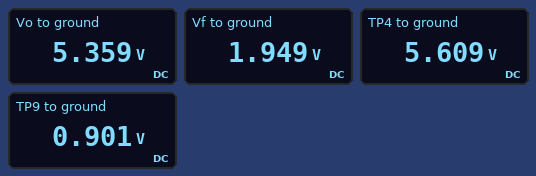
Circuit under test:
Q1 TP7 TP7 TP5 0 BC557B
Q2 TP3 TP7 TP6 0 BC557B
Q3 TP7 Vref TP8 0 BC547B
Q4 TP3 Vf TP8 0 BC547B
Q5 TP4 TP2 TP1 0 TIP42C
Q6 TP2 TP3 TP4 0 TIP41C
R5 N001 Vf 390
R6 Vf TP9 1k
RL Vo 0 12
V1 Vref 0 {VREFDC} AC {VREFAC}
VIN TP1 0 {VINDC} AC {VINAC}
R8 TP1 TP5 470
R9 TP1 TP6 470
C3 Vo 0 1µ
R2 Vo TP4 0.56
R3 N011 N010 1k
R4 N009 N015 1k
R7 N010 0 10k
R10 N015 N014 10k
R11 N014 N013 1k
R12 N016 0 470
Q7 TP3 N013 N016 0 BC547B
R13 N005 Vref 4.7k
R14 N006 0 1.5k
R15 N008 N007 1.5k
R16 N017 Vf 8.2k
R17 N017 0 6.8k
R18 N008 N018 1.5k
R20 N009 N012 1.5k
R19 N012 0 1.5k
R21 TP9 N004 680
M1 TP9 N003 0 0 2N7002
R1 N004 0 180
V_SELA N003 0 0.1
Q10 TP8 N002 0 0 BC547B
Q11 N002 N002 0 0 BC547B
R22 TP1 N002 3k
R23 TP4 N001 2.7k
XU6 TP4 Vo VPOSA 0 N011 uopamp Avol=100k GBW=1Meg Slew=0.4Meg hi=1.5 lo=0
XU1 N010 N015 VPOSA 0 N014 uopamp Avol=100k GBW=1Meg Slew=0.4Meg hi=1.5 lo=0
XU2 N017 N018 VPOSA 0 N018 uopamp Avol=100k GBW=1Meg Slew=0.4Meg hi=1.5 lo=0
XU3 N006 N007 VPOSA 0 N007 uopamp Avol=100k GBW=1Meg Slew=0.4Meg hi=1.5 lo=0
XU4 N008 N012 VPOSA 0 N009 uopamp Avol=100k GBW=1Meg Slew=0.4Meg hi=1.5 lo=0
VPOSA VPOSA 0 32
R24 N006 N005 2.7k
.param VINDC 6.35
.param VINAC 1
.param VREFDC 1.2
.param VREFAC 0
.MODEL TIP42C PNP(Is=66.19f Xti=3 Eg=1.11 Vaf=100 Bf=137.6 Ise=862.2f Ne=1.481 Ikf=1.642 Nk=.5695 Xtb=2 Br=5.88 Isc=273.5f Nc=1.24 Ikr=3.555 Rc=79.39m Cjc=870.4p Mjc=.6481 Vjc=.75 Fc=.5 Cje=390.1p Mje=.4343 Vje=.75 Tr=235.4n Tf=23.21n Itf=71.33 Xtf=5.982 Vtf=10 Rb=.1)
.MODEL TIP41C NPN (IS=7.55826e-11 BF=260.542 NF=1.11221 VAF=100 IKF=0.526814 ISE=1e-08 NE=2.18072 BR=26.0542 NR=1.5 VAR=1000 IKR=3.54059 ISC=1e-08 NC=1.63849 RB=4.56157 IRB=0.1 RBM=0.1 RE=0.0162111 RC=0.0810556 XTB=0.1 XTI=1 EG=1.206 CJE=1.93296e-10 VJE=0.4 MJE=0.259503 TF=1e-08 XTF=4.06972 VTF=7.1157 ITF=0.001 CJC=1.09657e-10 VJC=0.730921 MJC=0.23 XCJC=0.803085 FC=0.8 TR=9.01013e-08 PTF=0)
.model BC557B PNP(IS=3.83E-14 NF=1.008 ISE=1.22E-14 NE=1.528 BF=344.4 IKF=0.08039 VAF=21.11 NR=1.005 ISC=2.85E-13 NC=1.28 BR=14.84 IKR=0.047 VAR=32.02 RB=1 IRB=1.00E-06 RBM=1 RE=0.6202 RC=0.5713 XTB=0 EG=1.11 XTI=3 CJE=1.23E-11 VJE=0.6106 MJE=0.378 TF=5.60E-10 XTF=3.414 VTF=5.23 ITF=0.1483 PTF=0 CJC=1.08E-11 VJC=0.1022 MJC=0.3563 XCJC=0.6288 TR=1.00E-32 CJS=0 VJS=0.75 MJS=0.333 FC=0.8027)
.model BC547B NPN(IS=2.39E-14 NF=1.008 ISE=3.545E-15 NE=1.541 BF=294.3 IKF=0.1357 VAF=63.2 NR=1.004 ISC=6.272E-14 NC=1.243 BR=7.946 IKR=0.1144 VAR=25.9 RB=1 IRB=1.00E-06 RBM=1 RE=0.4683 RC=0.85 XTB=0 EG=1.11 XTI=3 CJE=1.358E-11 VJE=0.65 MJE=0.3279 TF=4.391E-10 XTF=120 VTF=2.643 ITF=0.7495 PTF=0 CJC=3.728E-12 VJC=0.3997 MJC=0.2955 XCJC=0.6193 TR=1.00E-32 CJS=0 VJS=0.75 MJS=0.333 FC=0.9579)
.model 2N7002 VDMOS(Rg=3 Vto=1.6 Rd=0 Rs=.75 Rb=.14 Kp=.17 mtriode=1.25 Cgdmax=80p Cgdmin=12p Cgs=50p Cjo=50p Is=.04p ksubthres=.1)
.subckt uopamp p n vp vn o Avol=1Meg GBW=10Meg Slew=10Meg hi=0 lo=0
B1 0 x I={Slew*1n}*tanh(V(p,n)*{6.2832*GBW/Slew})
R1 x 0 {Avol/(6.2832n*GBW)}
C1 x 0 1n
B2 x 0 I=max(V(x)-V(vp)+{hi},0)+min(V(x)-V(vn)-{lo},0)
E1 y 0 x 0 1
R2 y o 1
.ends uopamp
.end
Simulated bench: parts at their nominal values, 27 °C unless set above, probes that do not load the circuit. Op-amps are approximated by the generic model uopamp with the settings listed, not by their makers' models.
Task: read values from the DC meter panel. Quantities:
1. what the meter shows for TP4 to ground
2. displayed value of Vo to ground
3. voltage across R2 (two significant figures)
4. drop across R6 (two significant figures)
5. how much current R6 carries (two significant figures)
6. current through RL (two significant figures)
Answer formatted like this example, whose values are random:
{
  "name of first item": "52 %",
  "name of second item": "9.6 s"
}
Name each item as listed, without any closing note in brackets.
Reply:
{
  "what the meter shows for TP4 to ground": "5.609 V",
  "displayed value of Vo to ground": "5.359 V",
  "voltage across R2": "250 mV",
  "drop across R6": "1.0 V",
  "how much current R6 carries": "1.0 mA",
  "current through RL": "450 mA"
}
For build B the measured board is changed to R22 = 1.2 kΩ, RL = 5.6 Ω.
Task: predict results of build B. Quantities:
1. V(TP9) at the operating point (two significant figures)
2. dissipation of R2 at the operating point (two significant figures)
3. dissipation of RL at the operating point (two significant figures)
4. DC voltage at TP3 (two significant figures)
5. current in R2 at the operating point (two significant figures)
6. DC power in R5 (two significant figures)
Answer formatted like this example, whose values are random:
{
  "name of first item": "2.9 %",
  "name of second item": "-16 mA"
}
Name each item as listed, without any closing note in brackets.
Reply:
{
  "V(TP9) at the operating point": "890 mV",
  "dissipation of R2 at the operating point": "460 mW",
  "dissipation of RL at the operating point": "4.6 W",
  "DC voltage at TP3": "6.1 V",
  "current in R2 at the operating point": "900 mA",
  "DC power in R5": "540 µW"
}
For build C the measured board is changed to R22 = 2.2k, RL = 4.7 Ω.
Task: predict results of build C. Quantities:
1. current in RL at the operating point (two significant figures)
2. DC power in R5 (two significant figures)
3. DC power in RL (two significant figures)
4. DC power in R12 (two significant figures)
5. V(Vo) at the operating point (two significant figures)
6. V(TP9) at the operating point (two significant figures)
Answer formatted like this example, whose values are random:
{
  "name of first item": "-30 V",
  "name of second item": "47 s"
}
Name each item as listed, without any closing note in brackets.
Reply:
{
  "current in RL at the operating point": "1.1 A",
  "DC power in R5": "540 µW",
  "DC power in RL": "5.2 W",
  "DC power in R12": "80 mW",
  "V(Vo) at the operating point": "5.0 V",
  "V(TP9) at the operating point": "890 mV"
}
